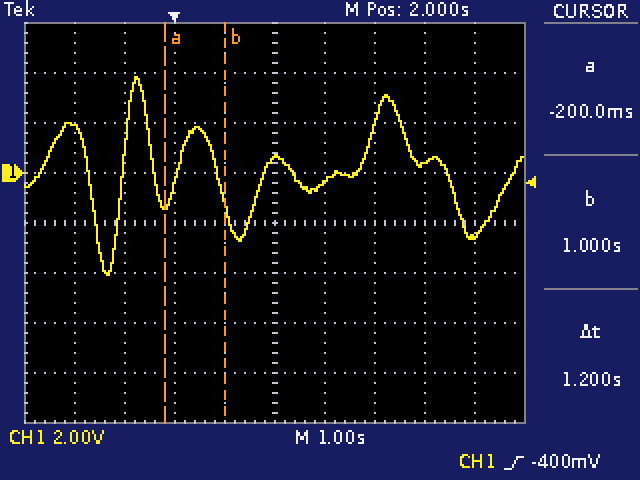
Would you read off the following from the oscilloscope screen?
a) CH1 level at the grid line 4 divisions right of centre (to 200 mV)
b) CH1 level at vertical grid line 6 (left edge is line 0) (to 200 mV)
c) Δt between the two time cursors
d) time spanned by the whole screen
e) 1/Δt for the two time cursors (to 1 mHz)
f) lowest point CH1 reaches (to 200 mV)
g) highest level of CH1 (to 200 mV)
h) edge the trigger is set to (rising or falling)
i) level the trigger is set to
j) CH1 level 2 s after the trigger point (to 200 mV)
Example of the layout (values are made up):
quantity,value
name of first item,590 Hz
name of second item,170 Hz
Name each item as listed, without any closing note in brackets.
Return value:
quantity,value
CH1 level at the grid line 4 divisions right of centre,-2.6 V
CH1 level at vertical grid line 6 (left edge is line 0),-400 mV
Δt between the two time cursors,1.2 s
time spanned by the whole screen,10 s
1/Δt for the two time cursors,833 mHz
lowest point CH1 reaches,-4.0 V
highest level of CH1,3.8 V
edge the trigger is set to,rising
level the trigger is set to,-400 mV
CH1 level 2 s after the trigger point,600 mV
